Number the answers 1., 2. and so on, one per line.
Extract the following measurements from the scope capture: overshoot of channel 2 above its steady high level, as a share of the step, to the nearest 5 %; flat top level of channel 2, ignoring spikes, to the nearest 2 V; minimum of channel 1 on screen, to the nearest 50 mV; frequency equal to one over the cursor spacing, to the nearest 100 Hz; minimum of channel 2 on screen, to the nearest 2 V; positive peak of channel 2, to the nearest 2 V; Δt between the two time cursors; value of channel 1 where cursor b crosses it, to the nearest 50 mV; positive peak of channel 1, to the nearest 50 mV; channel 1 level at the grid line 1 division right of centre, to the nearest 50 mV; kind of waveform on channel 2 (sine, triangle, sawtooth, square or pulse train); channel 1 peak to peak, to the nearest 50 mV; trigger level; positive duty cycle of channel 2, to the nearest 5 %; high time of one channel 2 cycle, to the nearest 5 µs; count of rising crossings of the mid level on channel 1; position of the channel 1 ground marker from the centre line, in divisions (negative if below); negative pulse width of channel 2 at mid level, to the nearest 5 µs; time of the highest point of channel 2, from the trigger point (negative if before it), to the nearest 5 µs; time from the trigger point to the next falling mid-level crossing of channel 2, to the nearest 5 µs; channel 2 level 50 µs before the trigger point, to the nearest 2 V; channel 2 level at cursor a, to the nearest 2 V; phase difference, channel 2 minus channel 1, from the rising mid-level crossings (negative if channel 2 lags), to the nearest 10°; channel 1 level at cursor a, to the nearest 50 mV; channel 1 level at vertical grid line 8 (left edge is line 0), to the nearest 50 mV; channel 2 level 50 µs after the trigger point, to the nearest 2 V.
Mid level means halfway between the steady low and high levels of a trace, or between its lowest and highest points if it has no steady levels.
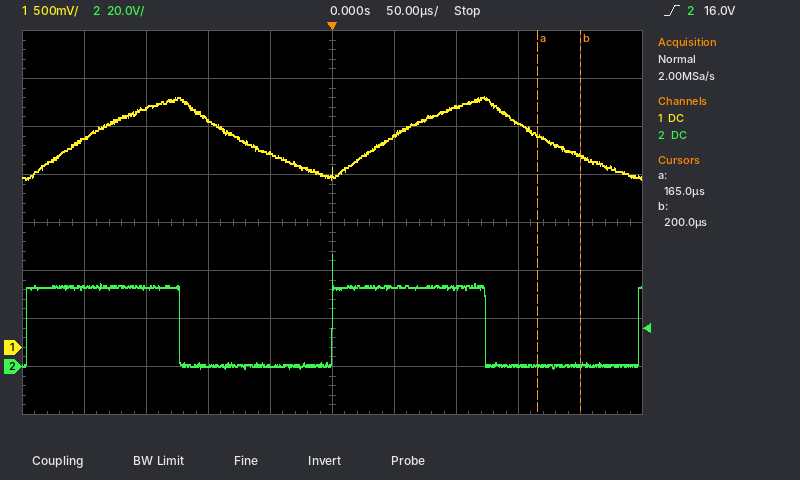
1. 40 %
2. 34 V
3. 1.75 V
4. 28.6 kHz
5. 0 V
6. 46 V
7. 35 µs
8. 2.00 V
9. 2.60 V
10. 2.20 V
11. square
12. 850 mV
13. 16.0 V
14. 50 %
15. 125 µs
16. 2
17. -2.6 div
18. 125 µs
19. 0 µs
20. 125 µs
21. 0 V
22. 0 V
23. +70°
24. 2.20 V
25. 2.35 V
26. 34 V
